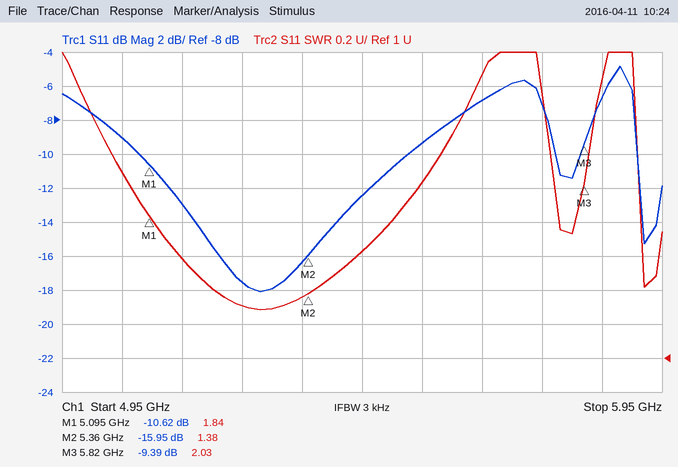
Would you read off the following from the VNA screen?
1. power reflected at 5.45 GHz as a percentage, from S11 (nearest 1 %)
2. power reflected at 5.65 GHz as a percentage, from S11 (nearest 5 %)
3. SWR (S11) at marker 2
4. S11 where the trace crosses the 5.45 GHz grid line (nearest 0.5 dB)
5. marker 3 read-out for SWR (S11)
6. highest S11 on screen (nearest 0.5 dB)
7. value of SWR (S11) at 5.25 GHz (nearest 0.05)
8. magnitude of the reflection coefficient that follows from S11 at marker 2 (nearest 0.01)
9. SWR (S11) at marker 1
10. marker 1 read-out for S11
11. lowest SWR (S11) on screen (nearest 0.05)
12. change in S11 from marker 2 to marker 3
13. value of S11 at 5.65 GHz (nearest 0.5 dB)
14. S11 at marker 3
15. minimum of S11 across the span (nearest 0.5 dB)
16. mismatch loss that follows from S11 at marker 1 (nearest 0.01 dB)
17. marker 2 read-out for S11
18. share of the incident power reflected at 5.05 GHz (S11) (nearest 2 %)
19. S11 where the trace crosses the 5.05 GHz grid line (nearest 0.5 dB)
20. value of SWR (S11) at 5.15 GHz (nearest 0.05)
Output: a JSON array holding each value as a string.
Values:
["6 %", "20 %", "1.38", "-12.5 dB", "2.03", "-5.0 dB", "1.30", "0.16", "1.84", "-10.62 dB", "1.30", "6.56 dB", "-7.0 dB", "-9.39 dB", "-18.0 dB", "0.39 dB", "-15.95 dB", "12 %", "-9.0 dB", "1.60"]
